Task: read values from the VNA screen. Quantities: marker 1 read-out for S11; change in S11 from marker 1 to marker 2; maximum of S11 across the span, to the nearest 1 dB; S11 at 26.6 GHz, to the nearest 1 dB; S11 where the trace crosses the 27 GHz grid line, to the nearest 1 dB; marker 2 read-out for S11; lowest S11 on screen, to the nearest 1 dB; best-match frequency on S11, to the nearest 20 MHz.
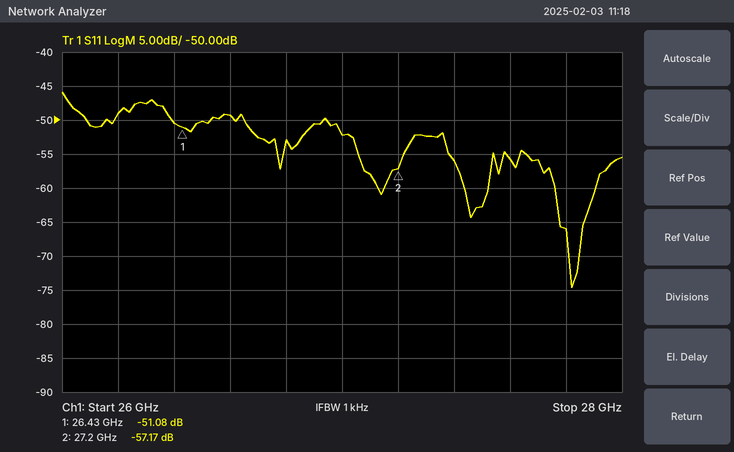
-51.08 dB
-6.09 dB
-46 dB
-49 dB
-52 dB
-57.17 dB
-75 dB
27.82 GHz
